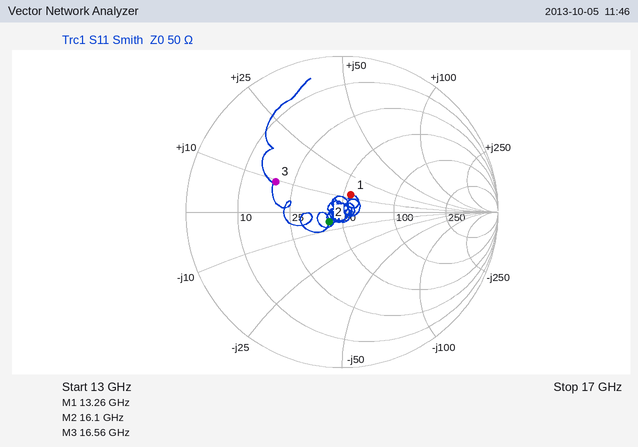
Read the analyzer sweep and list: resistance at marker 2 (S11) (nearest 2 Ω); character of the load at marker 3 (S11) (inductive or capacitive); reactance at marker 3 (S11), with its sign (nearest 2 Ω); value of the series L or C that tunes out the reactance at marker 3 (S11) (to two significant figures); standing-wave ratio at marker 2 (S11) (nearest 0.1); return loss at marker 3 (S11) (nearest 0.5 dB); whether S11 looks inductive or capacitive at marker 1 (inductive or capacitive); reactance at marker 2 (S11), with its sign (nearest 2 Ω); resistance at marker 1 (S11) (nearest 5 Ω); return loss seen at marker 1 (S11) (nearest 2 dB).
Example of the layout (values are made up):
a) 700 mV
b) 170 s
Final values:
a) 42 Ω
b) inductive
c) +10 Ω
d) 1.0 pF
e) 1.2
f) 6.5 dB
g) inductive
h) -6 Ω
i) 55 Ω
j) 18 dB
